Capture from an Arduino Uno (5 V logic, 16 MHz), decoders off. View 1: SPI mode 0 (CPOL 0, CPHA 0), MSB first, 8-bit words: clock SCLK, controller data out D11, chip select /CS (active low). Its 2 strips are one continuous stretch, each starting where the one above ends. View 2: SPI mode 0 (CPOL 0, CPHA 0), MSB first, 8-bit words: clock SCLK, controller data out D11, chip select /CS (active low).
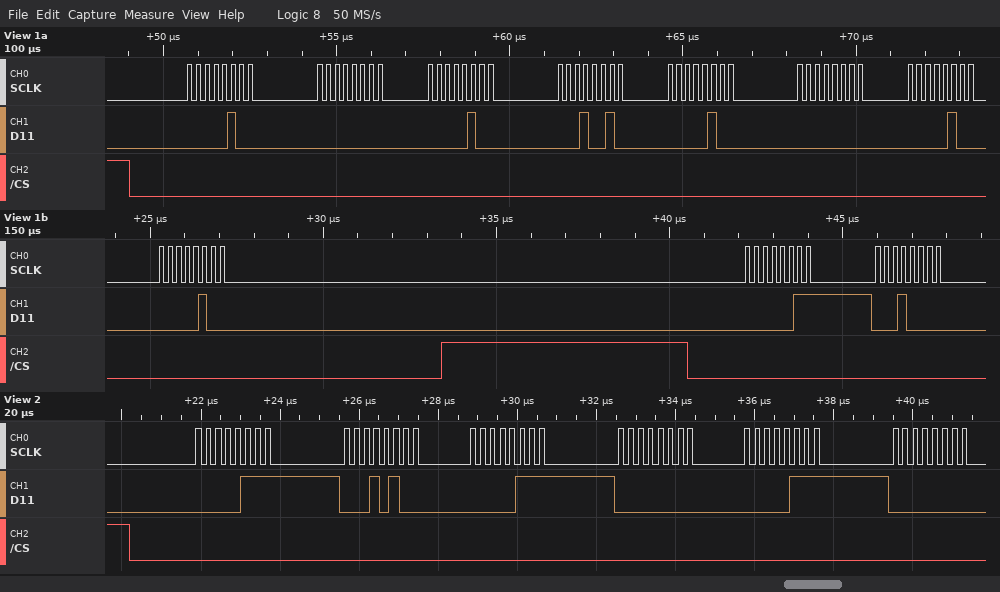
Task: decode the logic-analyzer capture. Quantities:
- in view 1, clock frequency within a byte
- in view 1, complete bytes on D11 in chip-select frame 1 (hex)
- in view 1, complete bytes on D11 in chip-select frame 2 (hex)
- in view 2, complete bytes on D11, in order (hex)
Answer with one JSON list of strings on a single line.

["4 MHz", "04 00 04 12 04 00 04 04", "03 10", "07 14 07 00 07 00"]
